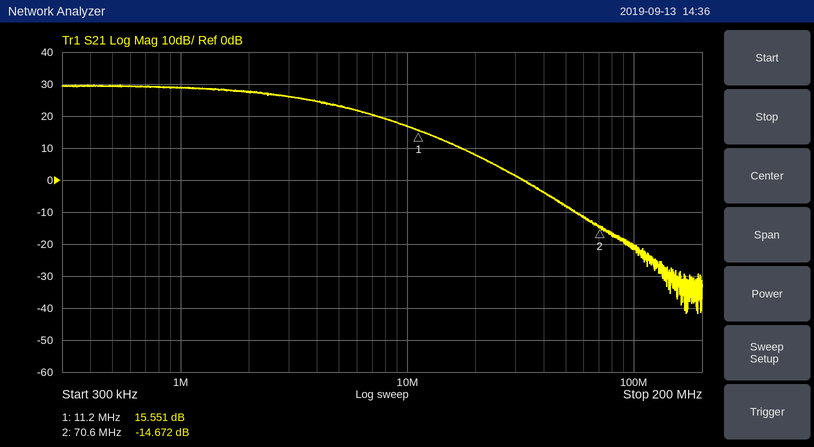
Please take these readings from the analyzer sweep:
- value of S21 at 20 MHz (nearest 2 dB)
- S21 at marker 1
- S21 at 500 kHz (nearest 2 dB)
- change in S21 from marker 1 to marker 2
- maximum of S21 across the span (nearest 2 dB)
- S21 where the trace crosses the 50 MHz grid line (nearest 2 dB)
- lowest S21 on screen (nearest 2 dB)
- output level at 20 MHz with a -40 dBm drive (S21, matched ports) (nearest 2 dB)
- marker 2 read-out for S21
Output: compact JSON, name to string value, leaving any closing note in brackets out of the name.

{"value of S21 at 20 MHz": "8 dB", "S21 at marker 1": "15.551 dB", "S21 at 500 kHz": "30 dB", "change in S21 from marker 1 to marker 2": "-30.223 dB", "maximum of S21 across the span": "30 dB", "S21 where the trace crosses the 50 MHz grid line": "-8 dB", "lowest S21 on screen": "-42 dB", "output level at 20 MHz with a -40 dBm drive (S21, matched ports)": "-32 dBm", "marker 2 read-out for S21": "-14.672 dB"}
